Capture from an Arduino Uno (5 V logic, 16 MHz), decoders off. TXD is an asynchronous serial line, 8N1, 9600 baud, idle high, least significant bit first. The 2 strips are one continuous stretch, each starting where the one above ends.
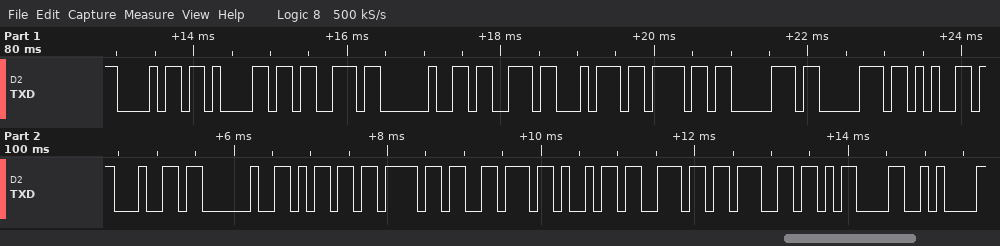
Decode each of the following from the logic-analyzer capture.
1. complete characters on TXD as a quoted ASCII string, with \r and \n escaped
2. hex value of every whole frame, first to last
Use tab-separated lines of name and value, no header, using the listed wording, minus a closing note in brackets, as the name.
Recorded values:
complete characters on TXD as a quoted ASCII string, with \r and \n escaped	"has stopped moving\r\n"
hex value of every whole frame, first to last	68 61 73 20 73 74 6F 70 70 65 64 20 6D 6F 76 69 6E 67 0D 0A
